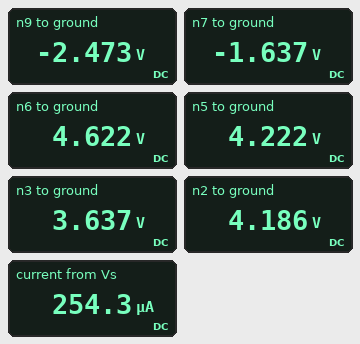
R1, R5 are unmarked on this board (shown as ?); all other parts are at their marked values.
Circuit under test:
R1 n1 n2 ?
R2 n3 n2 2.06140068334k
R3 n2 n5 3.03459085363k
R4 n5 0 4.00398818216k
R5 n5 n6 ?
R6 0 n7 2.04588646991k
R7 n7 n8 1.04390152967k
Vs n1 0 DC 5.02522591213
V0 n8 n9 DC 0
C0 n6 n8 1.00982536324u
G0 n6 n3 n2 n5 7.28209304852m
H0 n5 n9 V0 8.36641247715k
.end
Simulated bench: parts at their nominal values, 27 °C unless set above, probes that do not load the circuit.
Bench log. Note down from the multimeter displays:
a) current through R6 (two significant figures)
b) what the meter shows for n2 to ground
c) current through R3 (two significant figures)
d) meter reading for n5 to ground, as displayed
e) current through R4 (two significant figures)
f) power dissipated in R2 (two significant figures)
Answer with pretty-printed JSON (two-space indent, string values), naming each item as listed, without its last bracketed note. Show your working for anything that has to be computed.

{
  "current through R6": "(0 V - (-1.637 V)) / 2.046 kΩ = 800 µA",
  "what the meter shows for n2 to ground": "4.186 V",
  "current through R3": "(4.222 V - 4.186 V) / 3.035 kΩ = 12 µA",
  "meter reading for n5 to ground, as displayed": "4.222 V",
  "current through R4": "(4.222 V) / 4.004 kΩ = 1.1 mA",
  "power dissipated in R2": "(4.186 V - 3.637 V)^2 / 2.061 kΩ = 150 µW"
}
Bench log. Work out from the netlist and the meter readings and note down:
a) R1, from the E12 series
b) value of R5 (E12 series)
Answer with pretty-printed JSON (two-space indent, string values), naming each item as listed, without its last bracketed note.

{
  "R1, from the E12 series": "3.3 kΩ",
  "value of R5": "1.5 kΩ"
}
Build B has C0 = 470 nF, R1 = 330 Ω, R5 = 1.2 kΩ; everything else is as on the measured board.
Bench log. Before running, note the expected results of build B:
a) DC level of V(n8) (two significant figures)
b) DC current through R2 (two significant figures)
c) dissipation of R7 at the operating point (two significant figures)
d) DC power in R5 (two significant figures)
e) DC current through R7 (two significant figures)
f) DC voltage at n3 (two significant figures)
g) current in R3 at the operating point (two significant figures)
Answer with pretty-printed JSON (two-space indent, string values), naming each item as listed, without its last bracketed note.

{
  "DC level of V(n8)": "-2.9 V",
  "DC current through R2": "310 µA",
  "dissipation of R7 at the operating point": "930 µW",
  "DC power in R5": "120 µW",
  "DC current through R7": "940 µA",
  "DC voltage at n3": "4.3 V",
  "current in R3 at the operating point": "14 µA"
}
